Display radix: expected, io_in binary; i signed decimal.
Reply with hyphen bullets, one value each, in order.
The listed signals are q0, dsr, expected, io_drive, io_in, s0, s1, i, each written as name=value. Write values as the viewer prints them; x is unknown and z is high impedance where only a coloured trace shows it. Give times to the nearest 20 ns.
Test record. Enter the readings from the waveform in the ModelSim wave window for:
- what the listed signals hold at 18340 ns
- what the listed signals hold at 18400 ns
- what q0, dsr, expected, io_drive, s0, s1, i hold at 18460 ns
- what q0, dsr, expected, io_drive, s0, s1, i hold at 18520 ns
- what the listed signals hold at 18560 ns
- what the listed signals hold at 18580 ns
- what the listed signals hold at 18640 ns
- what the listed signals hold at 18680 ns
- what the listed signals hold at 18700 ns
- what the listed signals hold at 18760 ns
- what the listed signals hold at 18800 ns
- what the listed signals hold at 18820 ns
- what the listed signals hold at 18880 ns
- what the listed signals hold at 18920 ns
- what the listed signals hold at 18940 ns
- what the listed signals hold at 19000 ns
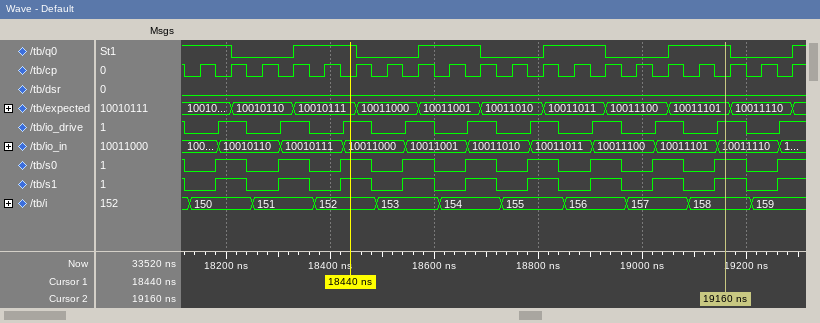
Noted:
- q0=1, dsr=0, expected=10010111, io_drive=1, io_in=10010111, s0=1, s1=1, i=151
- q0=1, dsr=0, expected=10010111, io_drive=0, io_in=10010111, s0=0, s1=0, i=152
- q0=0, dsr=0, expected=10011000, io_drive=1, s0=1, s1=1, i=152
- q0=0, dsr=0, expected=10011000, io_drive=0, s0=0, s1=0, i=153
- q0=0, dsr=0, expected=10011000, io_drive=1, io_in=10011001, s0=1, s1=1, i=153
- q0=1, dsr=0, expected=10011001, io_drive=1, io_in=10011001, s0=1, s1=1, i=153
- q0=1, dsr=0, expected=10011001, io_drive=0, io_in=10011001, s0=0, s1=0, i=154
- q0=1, dsr=0, expected=10011001, io_drive=1, io_in=10011010, s0=1, s1=1, i=154
- q0=0, dsr=0, expected=10011010, io_drive=1, io_in=10011010, s0=1, s1=1, i=154
- q0=0, dsr=0, expected=10011010, io_drive=0, io_in=10011010, s0=0, s1=0, i=155
- q0=0, dsr=0, expected=10011010, io_drive=1, io_in=10011011, s0=1, s1=1, i=155
- q0=1, dsr=0, expected=10011011, io_drive=1, io_in=10011011, s0=1, s1=1, i=155
- q0=1, dsr=0, expected=10011011, io_drive=0, io_in=10011011, s0=0, s1=0, i=156
- q0=1, dsr=0, expected=10011011, io_drive=1, io_in=10011100, s0=1, s1=1, i=156
- q0=0, dsr=0, expected=10011100, io_drive=1, io_in=10011100, s0=1, s1=1, i=156
- q0=0, dsr=0, expected=10011100, io_drive=0, io_in=10011100, s0=0, s1=0, i=157
